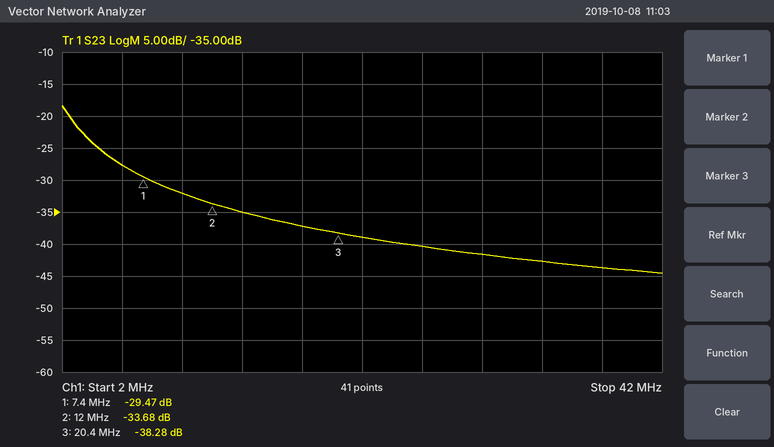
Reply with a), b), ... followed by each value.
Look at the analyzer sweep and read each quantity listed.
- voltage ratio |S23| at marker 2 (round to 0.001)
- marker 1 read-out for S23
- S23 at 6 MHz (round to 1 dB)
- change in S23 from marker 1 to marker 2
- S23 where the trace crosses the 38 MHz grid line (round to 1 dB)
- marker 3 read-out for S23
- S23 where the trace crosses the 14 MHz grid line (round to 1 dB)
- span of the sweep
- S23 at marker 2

a) 0.021
b) -29.47 dB
c) -28 dB
d) -4.21 dB
e) -44 dB
f) -38.28 dB
g) -35 dB
h) 40 MHz
i) -33.68 dB
